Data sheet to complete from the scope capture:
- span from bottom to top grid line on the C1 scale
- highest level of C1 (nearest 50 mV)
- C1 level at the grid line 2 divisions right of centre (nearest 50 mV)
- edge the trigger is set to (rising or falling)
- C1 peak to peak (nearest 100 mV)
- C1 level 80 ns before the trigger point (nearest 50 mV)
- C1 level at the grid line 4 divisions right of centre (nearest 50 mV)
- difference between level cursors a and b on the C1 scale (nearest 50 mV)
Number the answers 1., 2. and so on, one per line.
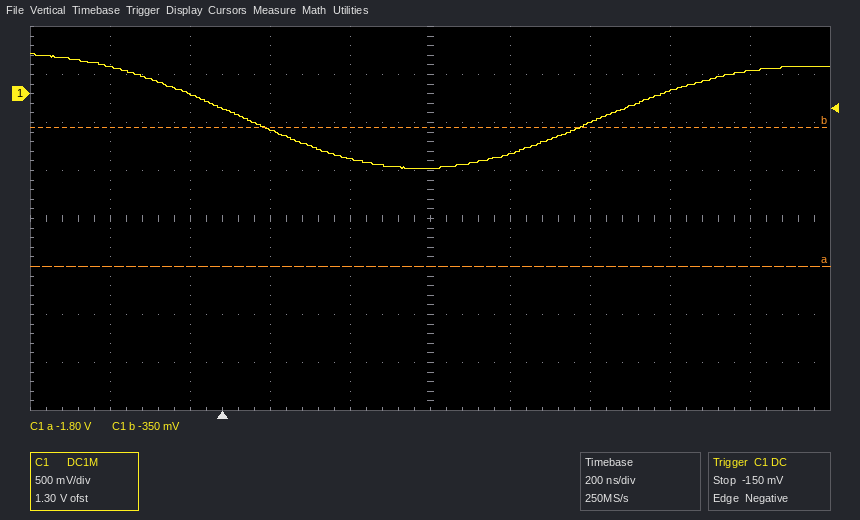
1. 4 V
2. 400 mV
3. -300 mV
4. falling
5. 1.20 V
6. 0 mV
7. 250 mV
8. 1.45 V
